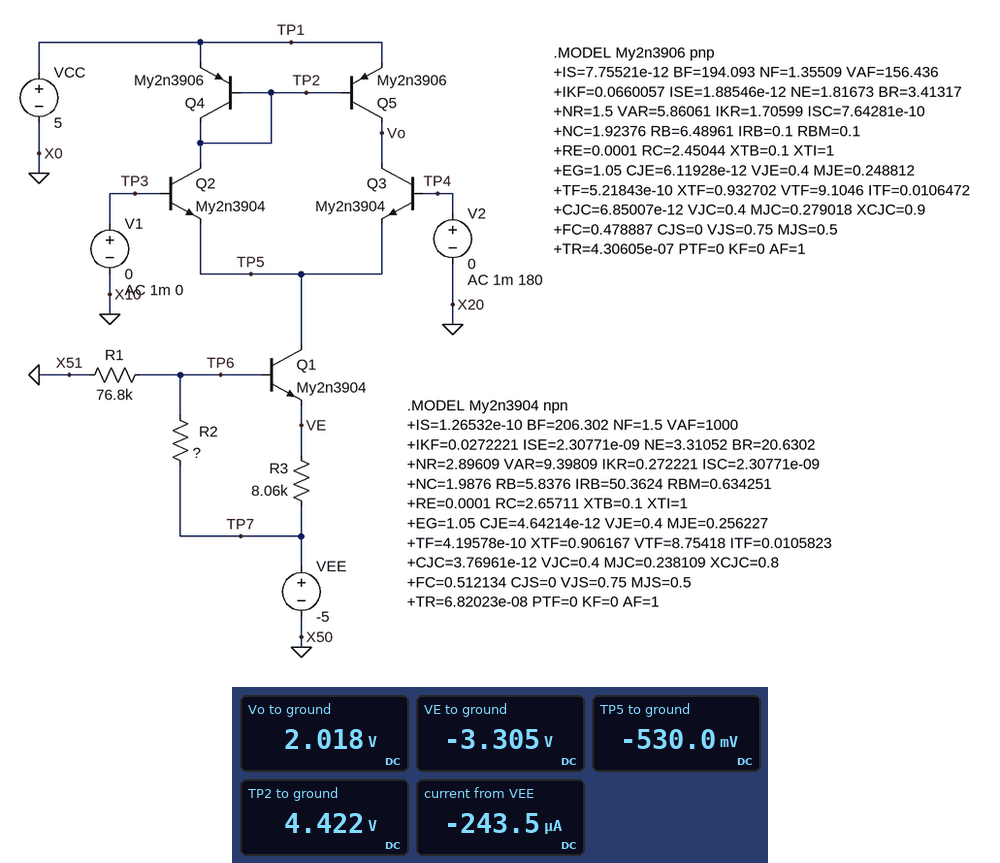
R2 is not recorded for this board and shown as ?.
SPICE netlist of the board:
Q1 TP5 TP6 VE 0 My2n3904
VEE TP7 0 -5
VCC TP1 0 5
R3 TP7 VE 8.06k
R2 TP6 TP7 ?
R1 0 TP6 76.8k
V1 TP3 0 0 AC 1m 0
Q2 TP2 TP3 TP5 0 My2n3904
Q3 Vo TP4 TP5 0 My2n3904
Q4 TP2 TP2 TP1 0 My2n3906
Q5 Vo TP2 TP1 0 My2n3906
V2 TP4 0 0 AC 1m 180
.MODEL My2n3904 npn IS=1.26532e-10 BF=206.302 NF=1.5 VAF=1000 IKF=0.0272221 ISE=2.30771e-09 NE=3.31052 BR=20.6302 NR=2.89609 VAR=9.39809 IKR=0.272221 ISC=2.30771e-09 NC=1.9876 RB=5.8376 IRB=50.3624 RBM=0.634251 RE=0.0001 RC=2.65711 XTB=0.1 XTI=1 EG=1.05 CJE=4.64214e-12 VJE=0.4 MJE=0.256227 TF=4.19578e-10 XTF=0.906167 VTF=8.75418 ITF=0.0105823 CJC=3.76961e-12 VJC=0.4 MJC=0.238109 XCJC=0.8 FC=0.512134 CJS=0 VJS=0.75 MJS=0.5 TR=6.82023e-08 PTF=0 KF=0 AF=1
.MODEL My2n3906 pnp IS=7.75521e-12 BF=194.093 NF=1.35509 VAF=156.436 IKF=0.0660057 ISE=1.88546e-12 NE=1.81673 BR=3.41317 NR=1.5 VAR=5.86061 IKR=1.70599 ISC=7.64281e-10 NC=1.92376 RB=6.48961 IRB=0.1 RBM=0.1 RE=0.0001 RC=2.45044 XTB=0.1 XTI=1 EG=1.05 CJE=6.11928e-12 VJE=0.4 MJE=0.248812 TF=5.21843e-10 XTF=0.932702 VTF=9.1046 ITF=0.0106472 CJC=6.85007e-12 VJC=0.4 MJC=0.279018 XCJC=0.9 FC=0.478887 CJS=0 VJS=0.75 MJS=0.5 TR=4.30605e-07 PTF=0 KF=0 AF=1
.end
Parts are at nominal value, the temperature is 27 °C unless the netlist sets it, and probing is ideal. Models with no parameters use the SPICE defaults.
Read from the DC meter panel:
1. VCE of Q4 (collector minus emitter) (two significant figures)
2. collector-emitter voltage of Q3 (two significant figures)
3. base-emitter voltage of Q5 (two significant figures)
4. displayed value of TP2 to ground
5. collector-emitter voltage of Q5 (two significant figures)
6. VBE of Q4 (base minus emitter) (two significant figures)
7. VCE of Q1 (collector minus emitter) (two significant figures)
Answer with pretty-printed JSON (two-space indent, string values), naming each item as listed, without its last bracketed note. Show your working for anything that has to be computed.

{
  "VCE of Q4 (collector minus emitter)": "4.422 V - 5 V = -580 mV",
  "collector-emitter voltage of Q3": "2.018 V - (-530 mV) = 2.5 V",
  "base-emitter voltage of Q5": "4.422 V - 5 V = -580 mV",
  "displayed value of TP2 to ground": "4.422 V",
  "collector-emitter voltage of Q5": "2.018 V - 5 V = -3.0 V",
  "VBE of Q4 (base minus emitter)": "4.422 V - 5 V = -580 mV",
  "VCE of Q1 (collector minus emitter)": "-530 mV - (-3.305 V) = 2.8 V"
}
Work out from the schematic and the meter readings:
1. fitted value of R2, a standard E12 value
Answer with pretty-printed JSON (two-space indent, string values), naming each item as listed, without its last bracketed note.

{
  "fitted value of R2, a standard E12 value": "68 kΩ"
}
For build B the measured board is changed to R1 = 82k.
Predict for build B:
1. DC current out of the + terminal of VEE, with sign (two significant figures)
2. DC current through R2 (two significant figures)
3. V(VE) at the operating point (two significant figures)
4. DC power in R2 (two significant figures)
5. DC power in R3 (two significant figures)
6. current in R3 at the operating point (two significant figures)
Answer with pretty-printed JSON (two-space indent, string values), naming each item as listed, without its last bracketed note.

{
  "DC current out of the + terminal of VEE, with sign": "-230 µA",
  "DC current through R2": "32 µA",
  "V(VE) at the operating point": "-3.4 V",
  "DC power in R2": "69 µW",
  "DC power in R3": "320 µW",
  "current in R3 at the operating point": "200 µA"
}
